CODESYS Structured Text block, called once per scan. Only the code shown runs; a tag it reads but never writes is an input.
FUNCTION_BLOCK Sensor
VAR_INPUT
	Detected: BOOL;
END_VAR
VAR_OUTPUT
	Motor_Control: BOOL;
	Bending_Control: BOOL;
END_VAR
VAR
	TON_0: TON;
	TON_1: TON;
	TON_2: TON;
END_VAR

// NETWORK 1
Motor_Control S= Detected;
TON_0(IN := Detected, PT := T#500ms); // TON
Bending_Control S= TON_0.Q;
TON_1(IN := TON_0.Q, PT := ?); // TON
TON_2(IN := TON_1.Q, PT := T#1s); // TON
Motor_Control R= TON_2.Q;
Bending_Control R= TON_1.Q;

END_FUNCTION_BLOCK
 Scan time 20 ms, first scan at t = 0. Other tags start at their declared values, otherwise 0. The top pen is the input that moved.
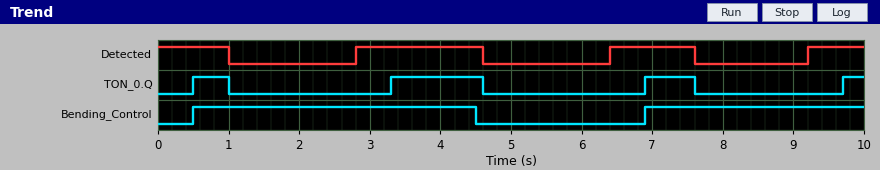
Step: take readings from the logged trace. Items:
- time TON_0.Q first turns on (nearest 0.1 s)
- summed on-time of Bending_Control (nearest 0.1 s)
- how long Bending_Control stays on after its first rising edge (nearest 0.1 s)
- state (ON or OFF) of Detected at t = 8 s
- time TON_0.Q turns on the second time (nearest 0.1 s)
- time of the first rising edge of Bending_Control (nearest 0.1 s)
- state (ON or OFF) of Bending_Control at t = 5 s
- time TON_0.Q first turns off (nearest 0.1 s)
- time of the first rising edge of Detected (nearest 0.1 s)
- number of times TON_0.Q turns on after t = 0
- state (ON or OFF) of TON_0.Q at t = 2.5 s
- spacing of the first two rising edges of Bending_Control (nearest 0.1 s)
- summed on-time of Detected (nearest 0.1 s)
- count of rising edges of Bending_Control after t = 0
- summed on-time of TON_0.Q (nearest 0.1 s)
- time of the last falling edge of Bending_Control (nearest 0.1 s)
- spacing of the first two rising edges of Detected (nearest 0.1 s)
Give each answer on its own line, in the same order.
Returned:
0.5 s
7.1 s
4.0 s
OFF
3.3 s
0.5 s
OFF
1.0 s
2.8 s
4
OFF
6.4 s
4.8 s
2
2.8 s
4.5 s
3.6 s
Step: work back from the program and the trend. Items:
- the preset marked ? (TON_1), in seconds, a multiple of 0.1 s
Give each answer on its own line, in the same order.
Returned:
1.2 s
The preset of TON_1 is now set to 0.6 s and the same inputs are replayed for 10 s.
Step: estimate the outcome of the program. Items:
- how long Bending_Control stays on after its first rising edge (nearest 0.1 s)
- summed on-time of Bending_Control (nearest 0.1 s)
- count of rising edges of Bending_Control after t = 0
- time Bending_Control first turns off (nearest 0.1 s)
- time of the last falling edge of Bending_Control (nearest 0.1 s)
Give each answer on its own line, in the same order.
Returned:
3.4 s
4.3 s
3
3.9 s
7.5 s
